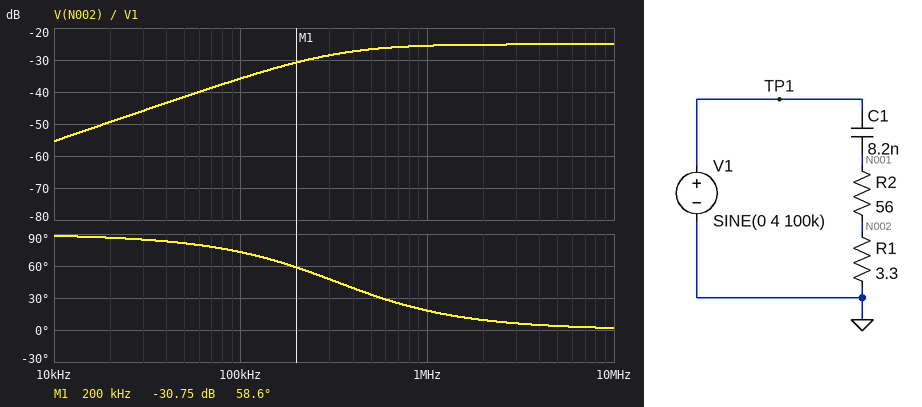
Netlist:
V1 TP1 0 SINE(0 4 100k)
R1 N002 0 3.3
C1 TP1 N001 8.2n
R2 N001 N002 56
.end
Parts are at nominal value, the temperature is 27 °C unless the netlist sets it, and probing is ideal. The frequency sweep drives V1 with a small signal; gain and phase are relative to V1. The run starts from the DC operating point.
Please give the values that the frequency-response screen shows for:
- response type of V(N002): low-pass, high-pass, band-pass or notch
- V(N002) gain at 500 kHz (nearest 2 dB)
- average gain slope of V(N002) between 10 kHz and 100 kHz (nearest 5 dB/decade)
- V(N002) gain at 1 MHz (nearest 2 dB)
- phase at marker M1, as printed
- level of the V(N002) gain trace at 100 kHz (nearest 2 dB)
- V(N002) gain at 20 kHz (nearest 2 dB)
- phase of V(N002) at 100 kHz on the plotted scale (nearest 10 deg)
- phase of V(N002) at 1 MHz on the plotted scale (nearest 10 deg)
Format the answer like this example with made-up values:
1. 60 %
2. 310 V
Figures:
1. high-pass
2. -26 dB
3. 20 dB/decade
4. -26 dB
5. 58.6 deg
6. -36 dB
7. -50 dB
8. 70 deg
9. 20 deg
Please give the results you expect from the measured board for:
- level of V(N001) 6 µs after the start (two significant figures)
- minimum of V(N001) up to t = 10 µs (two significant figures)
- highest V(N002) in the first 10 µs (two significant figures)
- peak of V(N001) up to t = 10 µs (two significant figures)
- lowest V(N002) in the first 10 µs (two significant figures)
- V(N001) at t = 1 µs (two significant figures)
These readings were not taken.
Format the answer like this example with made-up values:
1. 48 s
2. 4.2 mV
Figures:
1. -1.1 V
2. -1.2 V
3. 62 mV
4. 1.1 V
5. -65 mV
6. 960 mV
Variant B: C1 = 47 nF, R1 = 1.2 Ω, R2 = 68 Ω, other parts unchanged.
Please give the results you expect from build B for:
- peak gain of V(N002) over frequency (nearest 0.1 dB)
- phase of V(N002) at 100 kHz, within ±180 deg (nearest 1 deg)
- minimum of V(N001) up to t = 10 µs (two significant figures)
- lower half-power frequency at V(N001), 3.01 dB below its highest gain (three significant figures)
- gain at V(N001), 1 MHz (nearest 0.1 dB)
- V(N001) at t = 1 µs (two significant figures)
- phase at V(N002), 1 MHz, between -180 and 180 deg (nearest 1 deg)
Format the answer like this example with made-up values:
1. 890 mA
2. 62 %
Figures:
1. -35.2 dB
2. 26 deg
3. -3.8 V
4. 48.9 kHz
5. 0 dB
6. 2.0 V
7. 3 deg
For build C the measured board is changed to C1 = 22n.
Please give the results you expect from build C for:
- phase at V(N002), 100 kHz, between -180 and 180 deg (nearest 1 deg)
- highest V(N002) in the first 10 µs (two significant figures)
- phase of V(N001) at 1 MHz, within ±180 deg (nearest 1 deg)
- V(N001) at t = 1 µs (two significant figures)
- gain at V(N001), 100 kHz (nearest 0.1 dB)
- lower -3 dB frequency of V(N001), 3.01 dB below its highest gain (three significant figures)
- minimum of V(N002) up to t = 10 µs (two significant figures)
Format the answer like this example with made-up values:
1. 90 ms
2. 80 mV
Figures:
1. 51 deg
2. 110 mV
3. 7 deg
4. 1.6 V
5. -4.0 dB
6. 122 kHz
7. -140 mV
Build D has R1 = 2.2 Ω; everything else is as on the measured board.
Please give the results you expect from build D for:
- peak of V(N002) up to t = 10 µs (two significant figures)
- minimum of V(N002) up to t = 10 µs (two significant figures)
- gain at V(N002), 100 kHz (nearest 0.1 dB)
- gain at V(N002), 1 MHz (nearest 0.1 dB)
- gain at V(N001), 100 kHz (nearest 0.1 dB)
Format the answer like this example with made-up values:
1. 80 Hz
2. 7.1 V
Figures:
1. 42 mV
2. -43 mV
3. -39.3 dB
4. -28.9 dB
5. -10.8 dB
